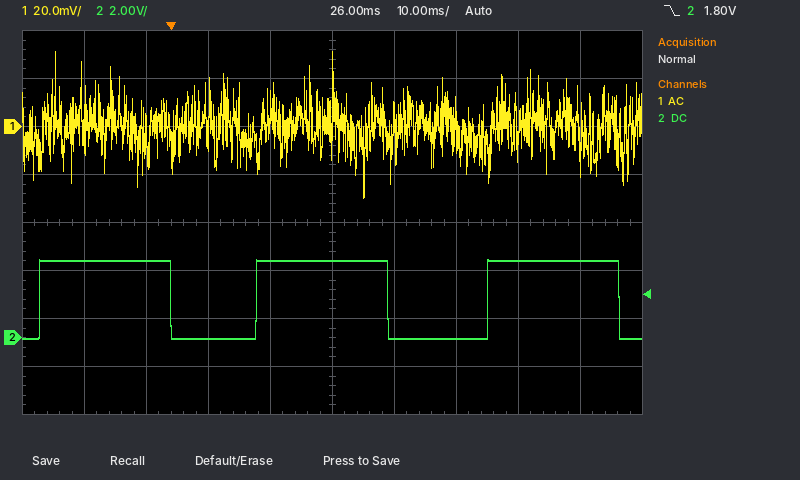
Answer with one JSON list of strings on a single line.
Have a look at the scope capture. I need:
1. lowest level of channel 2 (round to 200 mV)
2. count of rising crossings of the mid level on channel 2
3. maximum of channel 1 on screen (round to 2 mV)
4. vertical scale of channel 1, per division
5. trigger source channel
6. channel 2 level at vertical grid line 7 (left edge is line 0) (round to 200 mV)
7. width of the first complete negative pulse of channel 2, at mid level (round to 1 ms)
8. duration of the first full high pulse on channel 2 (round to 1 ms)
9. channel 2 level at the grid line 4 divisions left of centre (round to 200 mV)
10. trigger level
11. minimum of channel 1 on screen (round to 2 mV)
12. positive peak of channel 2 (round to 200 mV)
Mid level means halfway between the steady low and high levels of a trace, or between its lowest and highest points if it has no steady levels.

["0.0 V", "3", "32 mV", "20 mV", "channel 2", "0.0 V", "14 ms", "21 ms", "3.2 V", "1.80 V", "-30 mV", "3.2 V"]
